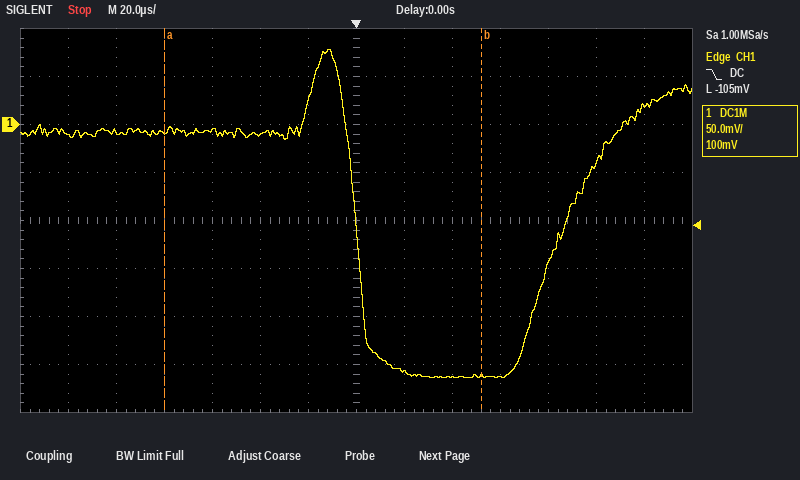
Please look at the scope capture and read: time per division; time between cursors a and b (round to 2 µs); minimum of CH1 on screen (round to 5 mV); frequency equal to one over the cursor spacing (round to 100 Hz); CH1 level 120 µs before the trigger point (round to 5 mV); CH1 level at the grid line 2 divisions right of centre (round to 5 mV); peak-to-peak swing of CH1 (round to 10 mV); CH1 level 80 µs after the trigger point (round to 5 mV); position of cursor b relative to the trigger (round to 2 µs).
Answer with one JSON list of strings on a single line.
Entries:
["20 µs", "132 µs", "-265 mV", "7.6 kHz", "-10 mV", "-265 mV", "340 mV", "-145 mV", "+52 µs"]
